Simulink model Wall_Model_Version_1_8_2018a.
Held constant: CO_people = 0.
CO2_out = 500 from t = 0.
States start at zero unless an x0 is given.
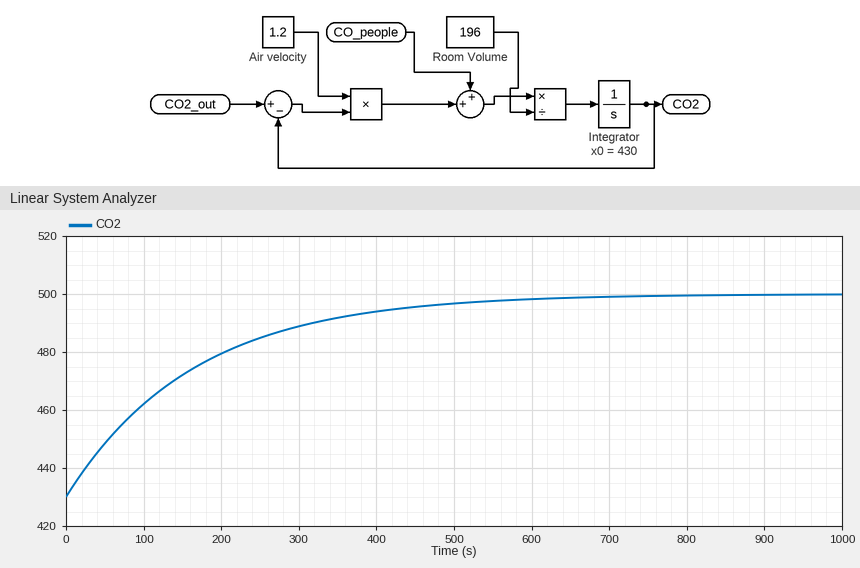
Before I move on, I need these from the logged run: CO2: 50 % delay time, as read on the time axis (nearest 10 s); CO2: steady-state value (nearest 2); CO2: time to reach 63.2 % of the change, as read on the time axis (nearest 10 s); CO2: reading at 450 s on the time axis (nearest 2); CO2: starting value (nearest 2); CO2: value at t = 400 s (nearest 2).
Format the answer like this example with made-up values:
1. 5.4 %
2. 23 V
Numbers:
1. 110 s
2. 500
3. 160 s
4. 496
5. 430
6. 494
